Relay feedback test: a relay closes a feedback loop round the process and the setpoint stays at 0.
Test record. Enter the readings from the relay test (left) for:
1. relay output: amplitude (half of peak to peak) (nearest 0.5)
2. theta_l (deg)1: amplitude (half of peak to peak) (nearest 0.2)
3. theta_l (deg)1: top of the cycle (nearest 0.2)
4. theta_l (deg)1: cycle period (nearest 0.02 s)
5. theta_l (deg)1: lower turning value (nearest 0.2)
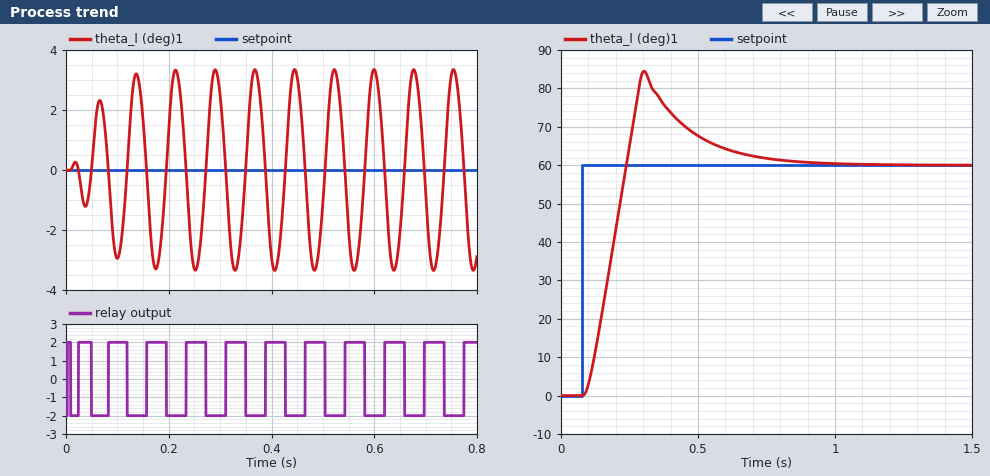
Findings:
2.0
3.4
3.4
0.08 s
-3.4
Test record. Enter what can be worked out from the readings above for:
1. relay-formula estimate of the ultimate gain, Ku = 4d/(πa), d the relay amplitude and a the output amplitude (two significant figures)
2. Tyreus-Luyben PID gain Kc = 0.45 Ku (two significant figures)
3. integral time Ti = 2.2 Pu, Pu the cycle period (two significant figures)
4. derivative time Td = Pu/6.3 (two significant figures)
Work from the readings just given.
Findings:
0.75
0.34
0.18 s
0.013 s
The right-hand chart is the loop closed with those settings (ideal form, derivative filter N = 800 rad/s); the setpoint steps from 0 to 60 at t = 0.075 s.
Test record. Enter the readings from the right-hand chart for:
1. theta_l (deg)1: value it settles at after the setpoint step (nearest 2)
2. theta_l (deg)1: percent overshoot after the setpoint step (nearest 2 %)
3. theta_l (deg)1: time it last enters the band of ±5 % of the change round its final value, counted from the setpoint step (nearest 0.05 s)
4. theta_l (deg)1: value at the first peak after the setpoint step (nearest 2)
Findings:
60
40 %
0.60 s
84
